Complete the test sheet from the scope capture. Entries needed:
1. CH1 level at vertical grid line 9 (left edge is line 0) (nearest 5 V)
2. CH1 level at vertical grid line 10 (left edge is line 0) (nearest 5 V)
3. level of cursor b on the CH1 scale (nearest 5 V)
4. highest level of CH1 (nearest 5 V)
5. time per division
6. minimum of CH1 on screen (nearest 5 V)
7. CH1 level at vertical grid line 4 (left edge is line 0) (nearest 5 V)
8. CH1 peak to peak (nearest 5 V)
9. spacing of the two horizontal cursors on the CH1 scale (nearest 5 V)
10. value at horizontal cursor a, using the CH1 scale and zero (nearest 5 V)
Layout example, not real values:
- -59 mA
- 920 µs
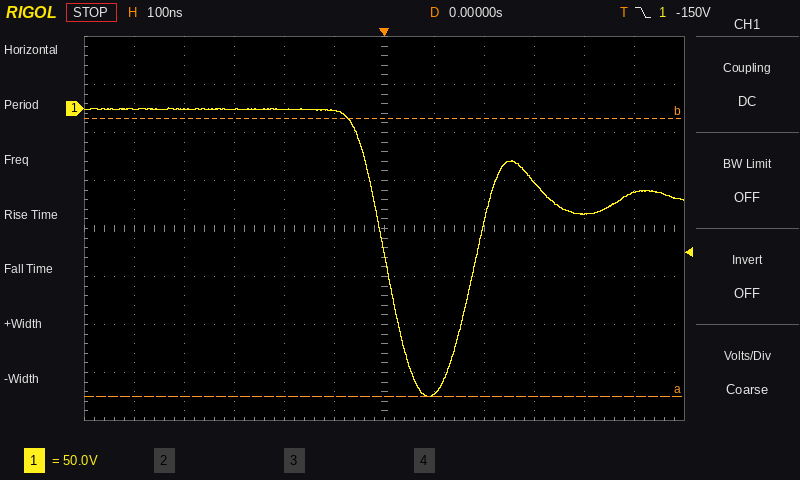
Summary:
- -75 V
- -110 V
- -10 V
- 0 V
- 100 ns
- -300 V
- 0 V
- 300 V
- 290 V
- -300 V
